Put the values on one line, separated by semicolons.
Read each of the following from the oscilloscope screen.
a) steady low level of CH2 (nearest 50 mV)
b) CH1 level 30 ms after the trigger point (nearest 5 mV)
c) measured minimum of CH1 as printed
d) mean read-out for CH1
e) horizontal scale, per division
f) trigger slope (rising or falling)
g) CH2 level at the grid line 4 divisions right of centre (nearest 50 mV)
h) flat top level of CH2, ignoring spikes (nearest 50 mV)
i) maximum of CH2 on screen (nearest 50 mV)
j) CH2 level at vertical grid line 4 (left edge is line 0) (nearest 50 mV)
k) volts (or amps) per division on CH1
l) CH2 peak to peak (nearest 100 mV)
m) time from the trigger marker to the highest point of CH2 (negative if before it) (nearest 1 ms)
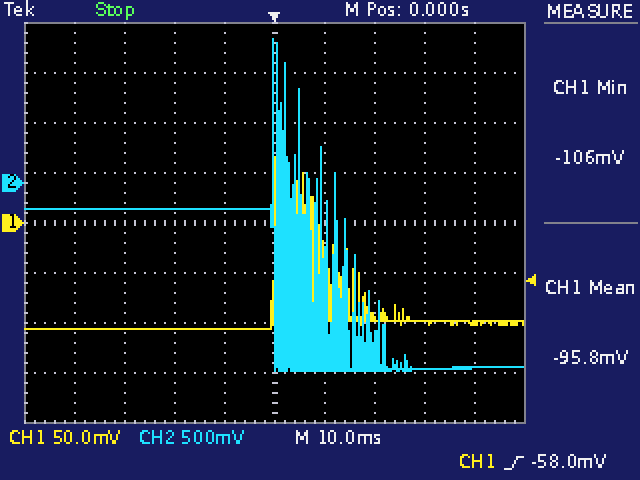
-1.85 V; -100 mV; -106 mV; -95.8 mV; 10 ms; rising; -1.85 V; -250 mV; 1.45 V; -250 mV; 50 mV; 3.30 V; 0 ms
